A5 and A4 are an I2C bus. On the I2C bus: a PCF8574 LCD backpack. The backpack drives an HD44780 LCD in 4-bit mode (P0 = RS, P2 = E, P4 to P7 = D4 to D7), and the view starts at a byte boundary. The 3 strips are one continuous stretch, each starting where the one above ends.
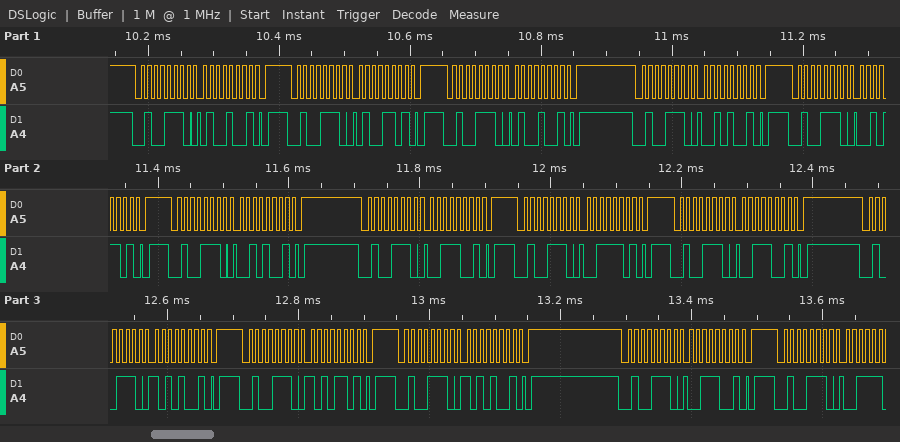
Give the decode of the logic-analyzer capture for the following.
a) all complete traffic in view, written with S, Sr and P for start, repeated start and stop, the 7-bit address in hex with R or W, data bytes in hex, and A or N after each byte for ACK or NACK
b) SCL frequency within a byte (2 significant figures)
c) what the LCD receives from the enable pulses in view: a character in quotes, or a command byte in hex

S 27W A 49 A P S 27W A 4D A P S 27W A 49 A P S 27W A 29 A P S 27W A 2D A P S 27W A 29 A P S 27W A 39 A P S 27W A 3D A P S 27W A 39 A P S 27W A A9 A P S 27W A AD A P S 27W A A9 A P S 27W A 39 A P S 27W A
100 kHz
'B' ':'
